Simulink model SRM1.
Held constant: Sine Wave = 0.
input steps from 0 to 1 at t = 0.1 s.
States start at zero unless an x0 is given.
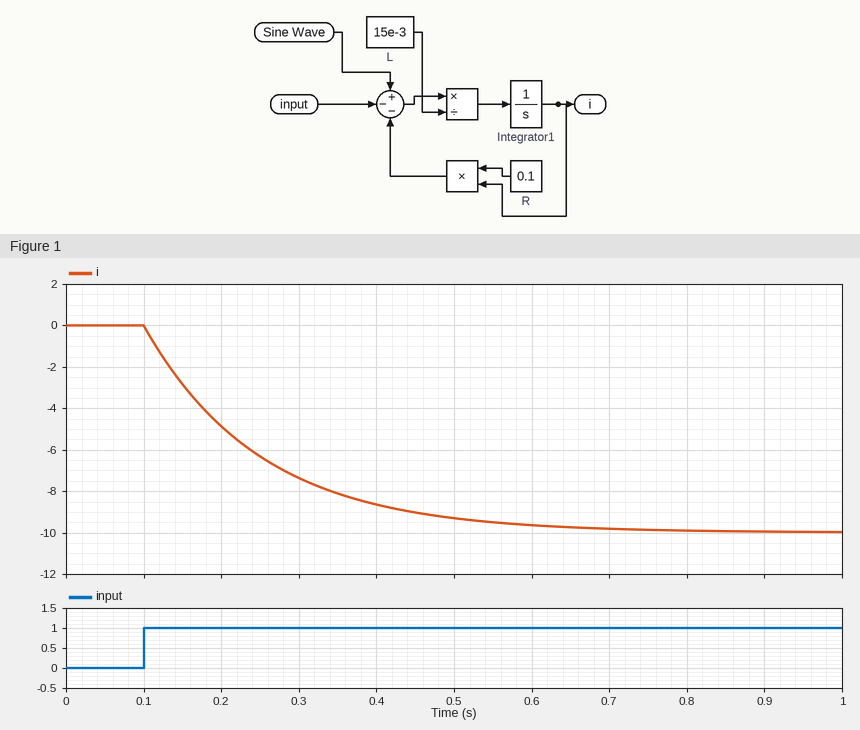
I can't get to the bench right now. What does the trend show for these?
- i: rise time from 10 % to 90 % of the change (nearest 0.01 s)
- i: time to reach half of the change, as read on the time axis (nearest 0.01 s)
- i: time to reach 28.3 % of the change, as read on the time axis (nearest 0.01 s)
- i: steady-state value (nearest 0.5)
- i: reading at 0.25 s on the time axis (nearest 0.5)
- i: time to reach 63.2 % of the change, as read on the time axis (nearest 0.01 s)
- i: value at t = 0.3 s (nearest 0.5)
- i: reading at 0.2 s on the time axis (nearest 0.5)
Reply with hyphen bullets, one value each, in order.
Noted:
- 0.33 s
- 0.20 s
- 0.15 s
- -10.0
- -6.5
- 0.25 s
- -7.5
- -5.0
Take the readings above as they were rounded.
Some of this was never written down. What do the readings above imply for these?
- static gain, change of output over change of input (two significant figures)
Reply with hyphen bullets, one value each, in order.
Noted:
- -10
